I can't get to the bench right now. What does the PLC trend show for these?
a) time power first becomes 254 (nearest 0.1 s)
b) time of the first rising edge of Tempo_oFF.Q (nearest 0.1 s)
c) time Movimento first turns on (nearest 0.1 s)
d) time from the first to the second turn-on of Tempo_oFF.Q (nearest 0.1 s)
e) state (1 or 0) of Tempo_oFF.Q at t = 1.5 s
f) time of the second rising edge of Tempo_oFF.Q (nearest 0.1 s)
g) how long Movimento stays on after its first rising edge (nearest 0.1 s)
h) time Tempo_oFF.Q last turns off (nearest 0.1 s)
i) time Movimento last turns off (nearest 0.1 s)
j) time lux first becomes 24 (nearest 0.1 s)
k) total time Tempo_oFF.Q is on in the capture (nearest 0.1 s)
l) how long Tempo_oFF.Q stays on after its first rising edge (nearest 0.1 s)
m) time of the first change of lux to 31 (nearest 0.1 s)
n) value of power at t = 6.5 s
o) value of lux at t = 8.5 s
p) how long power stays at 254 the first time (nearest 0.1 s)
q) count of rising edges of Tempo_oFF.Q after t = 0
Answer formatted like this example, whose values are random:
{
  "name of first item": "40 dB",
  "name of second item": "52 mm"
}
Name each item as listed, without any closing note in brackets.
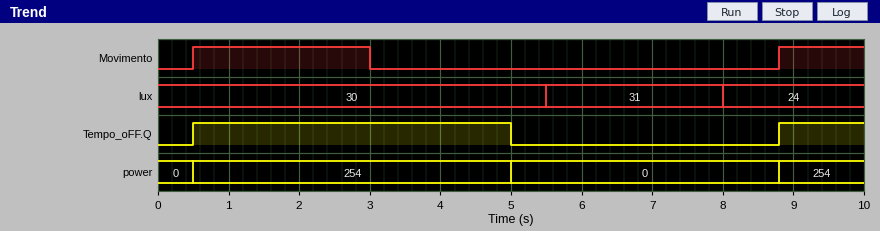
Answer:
{
  "time power first becomes 254": "0.5 s",
  "time of the first rising edge of Tempo_oFF.Q": "0.5 s",
  "time Movimento first turns on": "0.5 s",
  "time from the first to the second turn-on of Tempo_oFF.Q": "8.3 s",
  "state (1 or 0) of Tempo_oFF.Q at t = 1.5 s": "1",
  "time of the second rising edge of Tempo_oFF.Q": "8.8 s",
  "how long Movimento stays on after its first rising edge": "2.5 s",
  "time Tempo_oFF.Q last turns off": "5.0 s",
  "time Movimento last turns off": "3.0 s",
  "time lux first becomes 24": "8.0 s",
  "total time Tempo_oFF.Q is on in the capture": "5.7 s",
  "how long Tempo_oFF.Q stays on after its first rising edge": "4.5 s",
  "time of the first change of lux to 31": "5.5 s",
  "value of power at t = 6.5 s": "0",
  "value of lux at t = 8.5 s": "24",
  "how long power stays at 254 the first time": "4.5 s",
  "count of rising edges of Tempo_oFF.Q after t = 0": "2"
}
